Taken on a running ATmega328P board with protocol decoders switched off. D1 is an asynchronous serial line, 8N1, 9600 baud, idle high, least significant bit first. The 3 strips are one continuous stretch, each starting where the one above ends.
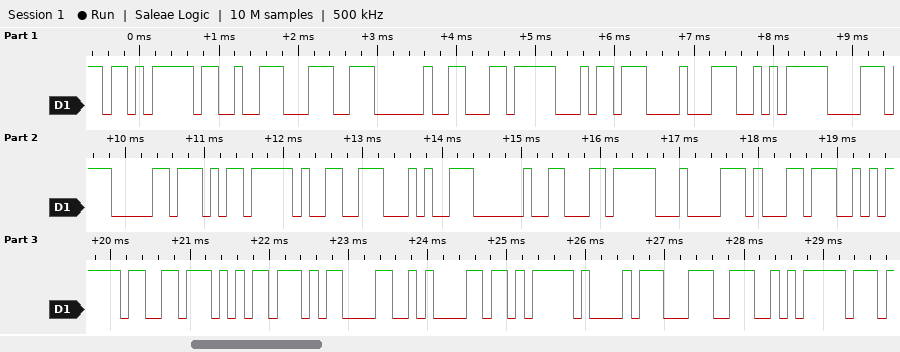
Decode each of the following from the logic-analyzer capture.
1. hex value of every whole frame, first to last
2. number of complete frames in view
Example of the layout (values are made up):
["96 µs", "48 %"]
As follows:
["EB 93 9C 20 EC B4 88 EA B8 B0 ED 99 94 20 EC 84 B1 EA B3 B5 0D 0A EB A1 9C EA", "26"]
